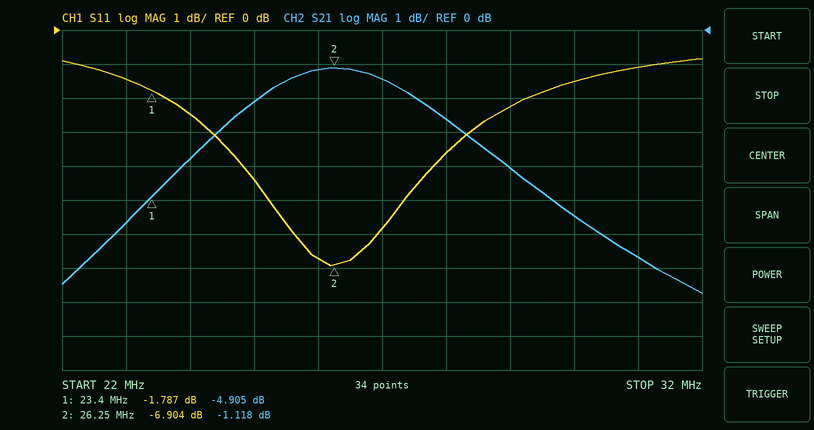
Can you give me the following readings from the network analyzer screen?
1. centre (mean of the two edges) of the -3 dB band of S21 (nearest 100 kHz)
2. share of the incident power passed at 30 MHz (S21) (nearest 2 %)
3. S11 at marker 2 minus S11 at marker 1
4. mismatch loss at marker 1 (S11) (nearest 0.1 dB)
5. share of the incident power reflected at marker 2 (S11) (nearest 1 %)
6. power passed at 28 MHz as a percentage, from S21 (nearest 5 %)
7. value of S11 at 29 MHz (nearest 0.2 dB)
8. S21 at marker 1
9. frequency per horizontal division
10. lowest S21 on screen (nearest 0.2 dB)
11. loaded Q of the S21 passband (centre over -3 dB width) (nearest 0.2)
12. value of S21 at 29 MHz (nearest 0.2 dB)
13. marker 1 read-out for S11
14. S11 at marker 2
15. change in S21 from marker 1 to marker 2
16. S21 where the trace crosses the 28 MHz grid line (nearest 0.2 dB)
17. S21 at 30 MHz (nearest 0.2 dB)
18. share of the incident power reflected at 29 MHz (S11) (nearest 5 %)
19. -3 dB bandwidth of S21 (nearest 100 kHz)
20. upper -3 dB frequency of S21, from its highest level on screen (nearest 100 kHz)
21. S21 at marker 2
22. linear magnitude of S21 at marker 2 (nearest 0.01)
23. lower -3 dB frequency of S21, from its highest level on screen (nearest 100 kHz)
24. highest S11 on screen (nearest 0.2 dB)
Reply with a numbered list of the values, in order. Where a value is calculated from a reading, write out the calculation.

1. 26.4 MHz
2. 10^(-5.4/10) ≈ 28.8 %, so 28 % to the nearest 2 %
3. -6.904 − (-1.787) = -5.117 dB
4. −10 log10(1 − 10^(-1.787/10)) ≈ 4.7 dB
5. 10^(-6.904/10) ≈ 20 %
6. 10^(-2.6/10) ≈ 55 %
7. -2.2 dB
8. -4.905 dB
9. 1 MHz
10. -7.8 dB
11. 26.4 MHz / 5.2 MHz ≈ 5.08, so 5.0 to the nearest 0.2
12. -4.0 dB
13. -1.787 dB
14. -6.904 dB
15. -1.118 − (-4.905) = 3.787 dB
16. -2.6 dB
17. -5.4 dB
18. 10^(-2.2/10) ≈ 60 %
19. 29.0 MHz − 23.8 MHz = 5.2 MHz
20. 29.0 MHz
21. -1.118 dB
22. 10^(-1.118/20) ≈ 0.88
23. 23.8 MHz
24. -0.8 dB
